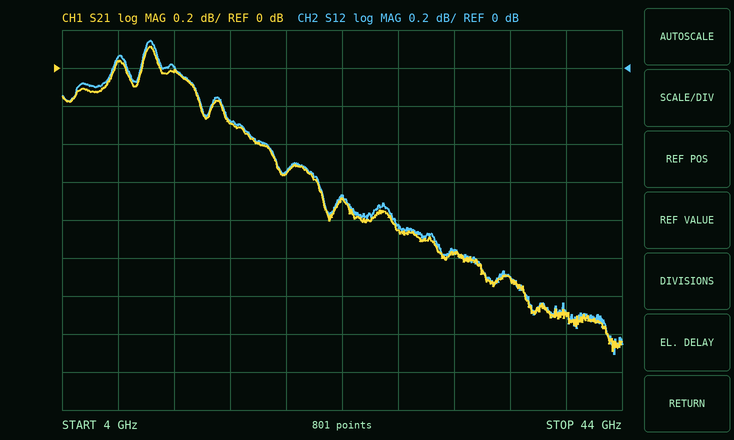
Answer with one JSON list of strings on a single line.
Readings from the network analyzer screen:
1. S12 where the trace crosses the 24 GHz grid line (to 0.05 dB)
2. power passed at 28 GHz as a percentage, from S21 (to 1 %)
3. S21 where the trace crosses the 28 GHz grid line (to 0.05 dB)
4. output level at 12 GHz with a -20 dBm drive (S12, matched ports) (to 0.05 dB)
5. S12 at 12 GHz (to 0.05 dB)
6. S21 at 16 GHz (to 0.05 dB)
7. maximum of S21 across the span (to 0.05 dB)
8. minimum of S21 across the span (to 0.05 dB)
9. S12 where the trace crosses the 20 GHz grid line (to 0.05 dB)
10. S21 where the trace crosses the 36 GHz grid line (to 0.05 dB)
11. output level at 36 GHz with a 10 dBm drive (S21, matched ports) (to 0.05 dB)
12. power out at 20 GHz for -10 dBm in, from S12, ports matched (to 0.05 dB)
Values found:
["-0.65 dB", "82 %", "-0.85 dB", "-20.00 dBm", "0.00 dB", "-0.30 dB", "0.10 dB", "-1.50 dB", "-0.55 dB", "-1.10 dB", "8.90 dBm", "-10.55 dBm"]
